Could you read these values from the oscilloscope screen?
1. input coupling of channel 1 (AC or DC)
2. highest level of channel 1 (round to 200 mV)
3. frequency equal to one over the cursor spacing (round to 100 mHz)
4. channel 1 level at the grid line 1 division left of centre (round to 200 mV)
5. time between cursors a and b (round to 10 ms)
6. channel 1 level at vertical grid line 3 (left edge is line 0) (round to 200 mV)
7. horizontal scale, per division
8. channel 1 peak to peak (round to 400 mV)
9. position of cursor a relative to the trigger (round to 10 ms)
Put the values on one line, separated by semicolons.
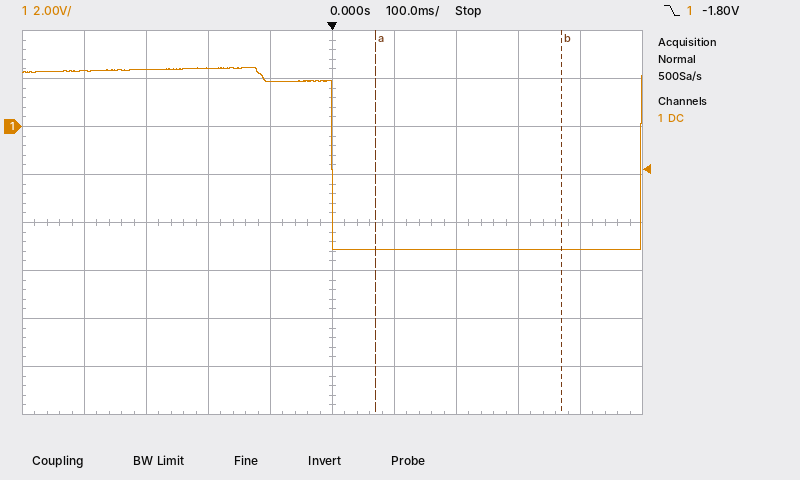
DC; 2.4 V; 3.3 Hz; 1.8 V; 300 ms; 2.4 V; 100 ms; 7.6 V; +70 ms
